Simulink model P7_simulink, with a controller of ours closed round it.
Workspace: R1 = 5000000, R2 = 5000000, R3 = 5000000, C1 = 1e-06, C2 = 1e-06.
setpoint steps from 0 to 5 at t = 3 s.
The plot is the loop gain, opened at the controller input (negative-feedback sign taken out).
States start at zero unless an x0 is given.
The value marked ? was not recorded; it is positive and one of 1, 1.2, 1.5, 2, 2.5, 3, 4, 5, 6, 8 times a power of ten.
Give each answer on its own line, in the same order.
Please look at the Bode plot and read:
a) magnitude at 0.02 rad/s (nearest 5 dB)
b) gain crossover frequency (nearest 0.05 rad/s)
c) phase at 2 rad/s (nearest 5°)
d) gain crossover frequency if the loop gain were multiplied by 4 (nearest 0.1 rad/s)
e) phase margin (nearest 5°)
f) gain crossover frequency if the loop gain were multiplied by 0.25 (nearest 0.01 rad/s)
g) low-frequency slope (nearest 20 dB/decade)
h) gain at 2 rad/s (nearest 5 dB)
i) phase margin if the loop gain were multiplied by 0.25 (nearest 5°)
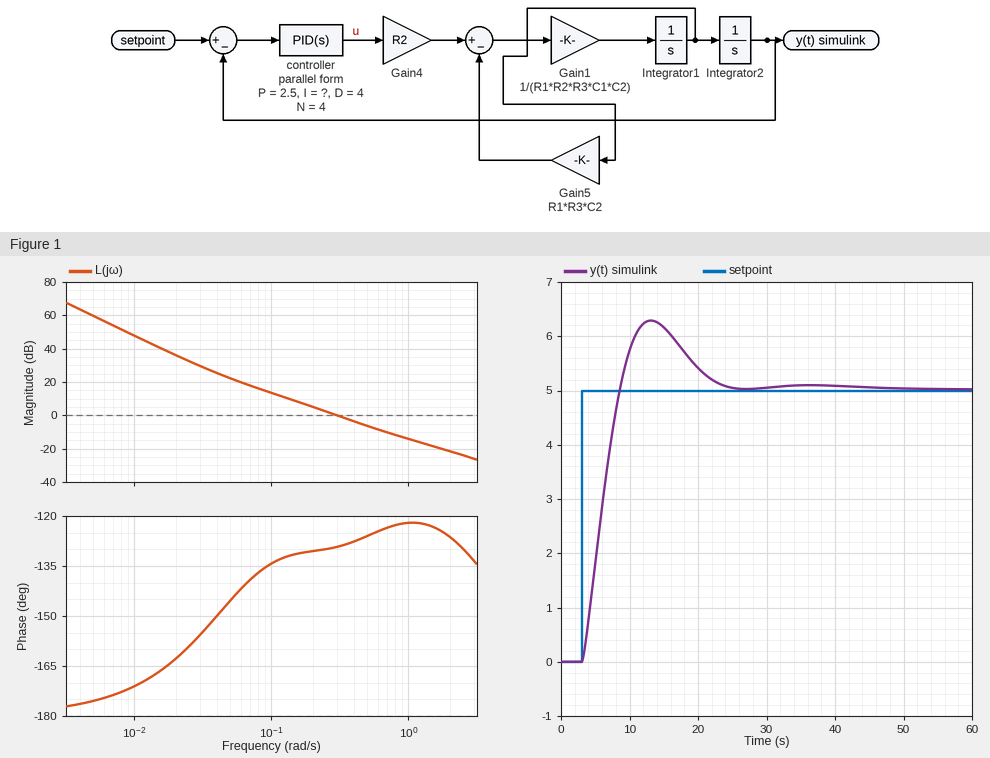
35 dB
0.30 rad/s
-125°
0.8 rad/s
50°
0.11 rad/s
-40 dB/decade
-20 dB
45°
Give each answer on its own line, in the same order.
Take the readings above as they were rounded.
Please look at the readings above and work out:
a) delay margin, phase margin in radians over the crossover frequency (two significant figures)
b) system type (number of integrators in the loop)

2.9 s
2
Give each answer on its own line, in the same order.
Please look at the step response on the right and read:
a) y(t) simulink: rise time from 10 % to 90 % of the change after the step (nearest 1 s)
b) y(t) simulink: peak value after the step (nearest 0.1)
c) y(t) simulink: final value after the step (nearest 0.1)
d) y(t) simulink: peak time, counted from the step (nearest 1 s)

4 s
6.3
5.0
10 s
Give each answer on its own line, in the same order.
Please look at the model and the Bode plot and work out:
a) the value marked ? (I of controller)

0.12
